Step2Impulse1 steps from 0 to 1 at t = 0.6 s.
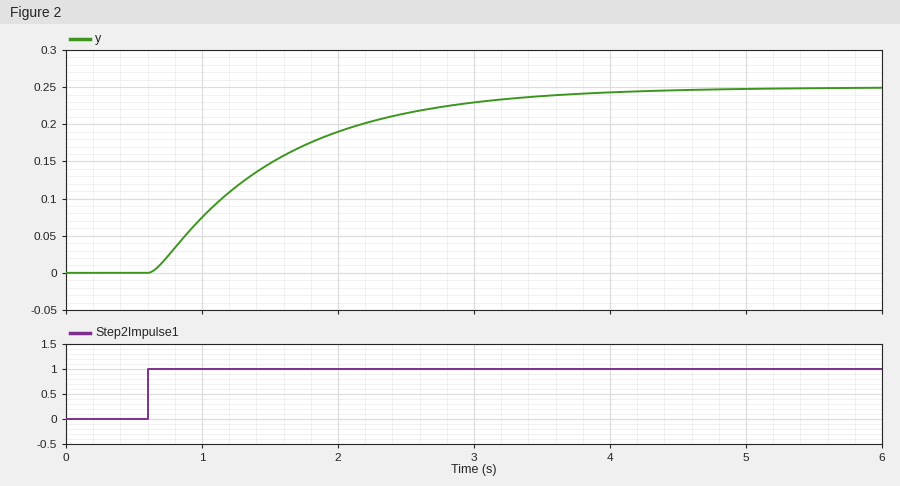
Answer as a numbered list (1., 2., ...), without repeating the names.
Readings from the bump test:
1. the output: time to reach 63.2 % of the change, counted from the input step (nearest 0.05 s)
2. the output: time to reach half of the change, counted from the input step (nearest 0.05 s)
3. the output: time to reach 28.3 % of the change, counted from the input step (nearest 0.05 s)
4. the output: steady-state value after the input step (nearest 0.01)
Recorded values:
1. 1.00 s
2. 0.70 s
3. 0.40 s
4. 0.25
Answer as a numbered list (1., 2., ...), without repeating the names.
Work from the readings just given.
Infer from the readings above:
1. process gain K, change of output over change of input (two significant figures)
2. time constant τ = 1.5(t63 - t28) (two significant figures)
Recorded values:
1. 0.25
2. 0.90 s
